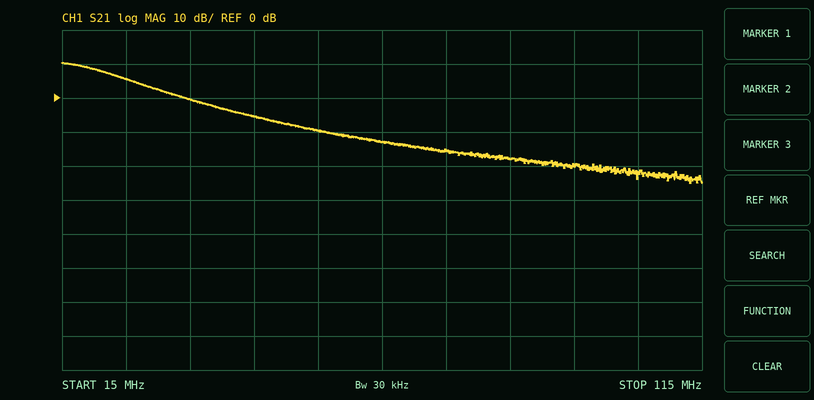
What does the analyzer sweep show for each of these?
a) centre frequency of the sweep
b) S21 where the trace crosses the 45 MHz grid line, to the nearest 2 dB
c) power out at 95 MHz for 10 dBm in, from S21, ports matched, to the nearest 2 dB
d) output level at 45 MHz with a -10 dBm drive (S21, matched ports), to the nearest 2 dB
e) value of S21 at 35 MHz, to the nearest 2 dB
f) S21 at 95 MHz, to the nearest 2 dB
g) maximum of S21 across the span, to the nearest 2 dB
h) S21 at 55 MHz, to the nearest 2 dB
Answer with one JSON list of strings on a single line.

["65 MHz", "-6 dB", "-10 dBm", "-16 dBm", "0 dB", "-20 dB", "10 dB", "-10 dB"]
